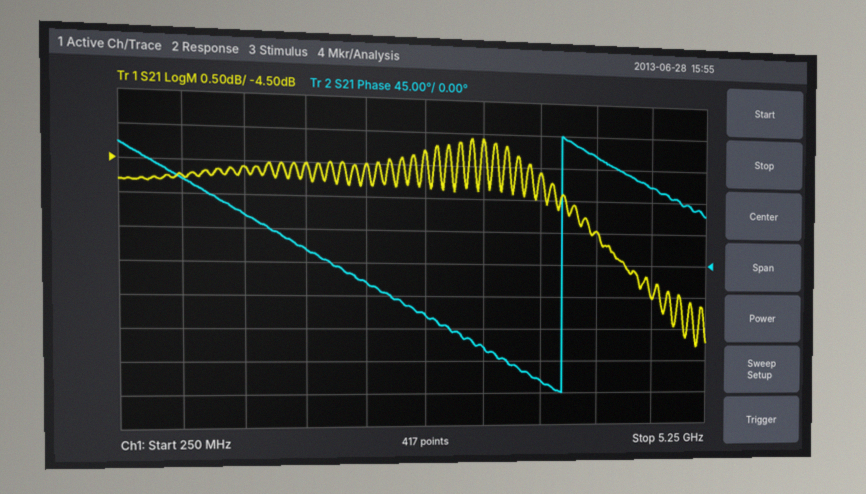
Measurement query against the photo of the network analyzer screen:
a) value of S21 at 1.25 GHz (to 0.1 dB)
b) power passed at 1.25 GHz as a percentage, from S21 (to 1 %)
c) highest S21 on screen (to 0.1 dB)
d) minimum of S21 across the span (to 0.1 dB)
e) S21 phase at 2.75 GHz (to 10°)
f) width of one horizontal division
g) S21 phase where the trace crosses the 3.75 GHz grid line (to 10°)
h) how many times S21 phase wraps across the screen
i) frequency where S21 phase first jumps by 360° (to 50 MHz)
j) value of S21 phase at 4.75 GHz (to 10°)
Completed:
-4.6 dB
35 %
-4.1 dB
-7.3 dB
-70°
500 MHz
-160°
1
3.95 GHz
110°
